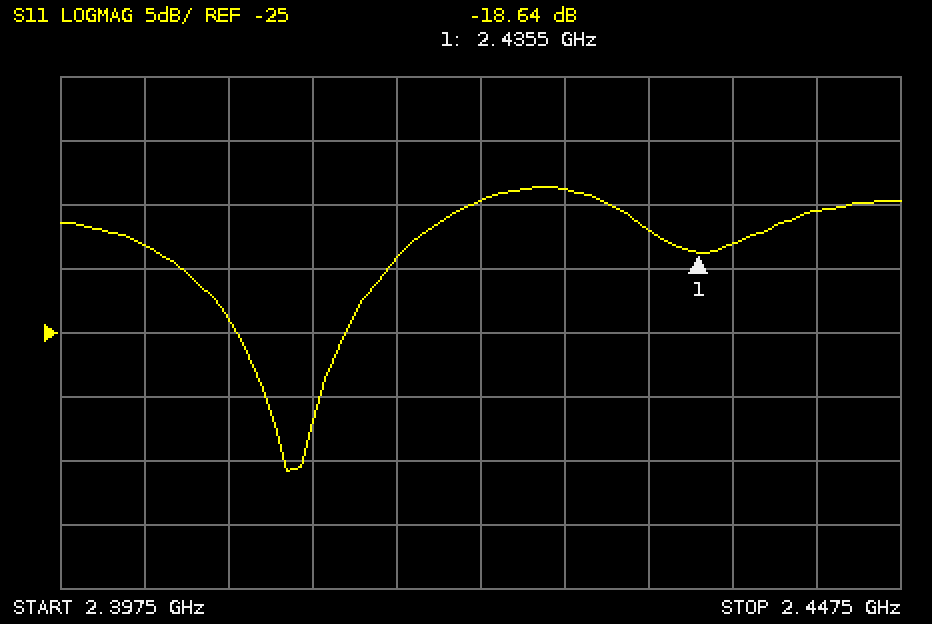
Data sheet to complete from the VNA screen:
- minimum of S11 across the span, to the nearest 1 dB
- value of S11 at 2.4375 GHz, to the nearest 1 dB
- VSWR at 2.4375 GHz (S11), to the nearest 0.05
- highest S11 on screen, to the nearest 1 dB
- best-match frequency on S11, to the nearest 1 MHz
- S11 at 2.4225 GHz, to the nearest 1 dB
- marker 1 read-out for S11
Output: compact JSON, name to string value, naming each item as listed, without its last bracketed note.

{"minimum of S11 across the span, to the nearest 1 dB": "-36 dB", "value of S11 at 2.4375 GHz, to the nearest 1 dB": "-18 dB", "VSWR at 2.4375 GHz (S11), to the nearest 0.05": "1.30", "highest S11 on screen, to the nearest 1 dB": "-14 dB", "best-match frequency on S11, to the nearest 1 MHz": "2.411 GHz", "S11 at 2.4225 GHz, to the nearest 1 dB": "-15 dB", "marker 1 read-out for S11": "-18.64 dB"}
